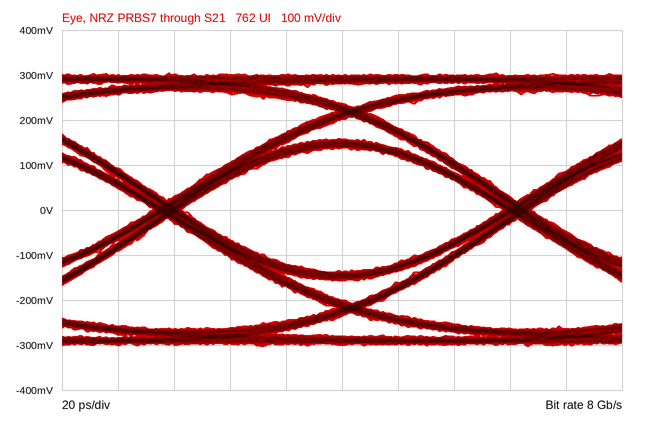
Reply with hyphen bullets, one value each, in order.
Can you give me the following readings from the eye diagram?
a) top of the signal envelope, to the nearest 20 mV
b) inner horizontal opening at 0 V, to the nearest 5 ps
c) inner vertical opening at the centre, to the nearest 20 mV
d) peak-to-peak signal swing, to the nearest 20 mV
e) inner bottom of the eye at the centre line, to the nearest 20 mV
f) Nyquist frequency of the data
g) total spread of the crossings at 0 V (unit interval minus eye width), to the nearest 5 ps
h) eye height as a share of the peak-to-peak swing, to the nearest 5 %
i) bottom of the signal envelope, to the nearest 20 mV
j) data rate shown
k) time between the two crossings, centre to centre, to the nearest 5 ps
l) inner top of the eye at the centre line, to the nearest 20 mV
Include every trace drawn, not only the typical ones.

- 300 mV
- 115 ps
- 280 mV
- 600 mV
- -140 mV
- 4 GHz
- 10 ps
- 45 %
- -300 mV
- 8 Gb/s
- 125 ps
- 140 mV
